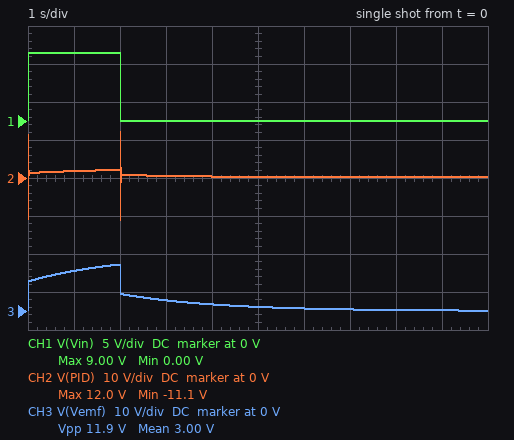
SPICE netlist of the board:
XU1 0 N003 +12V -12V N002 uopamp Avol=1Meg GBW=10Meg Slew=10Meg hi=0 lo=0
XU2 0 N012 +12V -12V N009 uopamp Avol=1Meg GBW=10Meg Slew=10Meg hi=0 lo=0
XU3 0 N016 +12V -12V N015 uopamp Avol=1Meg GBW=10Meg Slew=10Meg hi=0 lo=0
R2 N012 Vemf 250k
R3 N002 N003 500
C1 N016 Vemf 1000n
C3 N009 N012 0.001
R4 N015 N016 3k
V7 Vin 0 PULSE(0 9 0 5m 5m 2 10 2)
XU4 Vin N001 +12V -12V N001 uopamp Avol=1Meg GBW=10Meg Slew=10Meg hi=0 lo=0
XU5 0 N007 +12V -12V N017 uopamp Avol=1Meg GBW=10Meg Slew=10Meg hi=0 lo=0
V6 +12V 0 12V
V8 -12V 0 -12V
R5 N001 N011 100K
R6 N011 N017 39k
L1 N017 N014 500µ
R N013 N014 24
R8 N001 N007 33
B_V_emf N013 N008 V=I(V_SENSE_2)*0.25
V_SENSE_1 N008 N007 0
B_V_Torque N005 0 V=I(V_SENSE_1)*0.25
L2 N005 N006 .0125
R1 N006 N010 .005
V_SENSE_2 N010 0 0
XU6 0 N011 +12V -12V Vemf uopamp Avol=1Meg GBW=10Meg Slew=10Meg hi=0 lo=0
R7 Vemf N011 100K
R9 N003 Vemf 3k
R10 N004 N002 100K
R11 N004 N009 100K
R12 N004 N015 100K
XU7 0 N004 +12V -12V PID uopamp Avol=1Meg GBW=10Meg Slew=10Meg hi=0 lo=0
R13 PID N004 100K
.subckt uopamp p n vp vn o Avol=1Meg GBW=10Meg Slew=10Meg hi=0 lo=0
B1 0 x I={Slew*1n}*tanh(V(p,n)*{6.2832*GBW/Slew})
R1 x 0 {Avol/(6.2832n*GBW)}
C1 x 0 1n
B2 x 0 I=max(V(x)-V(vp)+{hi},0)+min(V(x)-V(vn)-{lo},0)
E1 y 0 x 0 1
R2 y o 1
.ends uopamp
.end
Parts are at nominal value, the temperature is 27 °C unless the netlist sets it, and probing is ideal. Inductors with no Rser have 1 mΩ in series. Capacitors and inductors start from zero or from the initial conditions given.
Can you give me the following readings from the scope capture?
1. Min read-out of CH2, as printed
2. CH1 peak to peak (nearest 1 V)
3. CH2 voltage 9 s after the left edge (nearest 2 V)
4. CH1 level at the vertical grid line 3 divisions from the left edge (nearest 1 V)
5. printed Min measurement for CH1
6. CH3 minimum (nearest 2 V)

-11.1 V
9 V
0 V
0 V
0.00 V
0 V
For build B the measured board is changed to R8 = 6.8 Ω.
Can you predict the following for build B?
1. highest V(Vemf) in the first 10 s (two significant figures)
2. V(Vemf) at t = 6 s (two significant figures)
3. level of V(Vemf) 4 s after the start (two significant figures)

12 V
1.4 V
3.7 V
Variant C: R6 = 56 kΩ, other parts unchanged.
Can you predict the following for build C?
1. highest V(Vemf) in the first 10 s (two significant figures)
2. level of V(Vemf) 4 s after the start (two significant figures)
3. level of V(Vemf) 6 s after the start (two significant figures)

5.8 V
1.2 V
460 mV
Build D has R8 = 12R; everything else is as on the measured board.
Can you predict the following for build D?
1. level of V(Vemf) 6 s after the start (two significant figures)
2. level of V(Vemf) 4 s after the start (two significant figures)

1.2 V
3.2 V
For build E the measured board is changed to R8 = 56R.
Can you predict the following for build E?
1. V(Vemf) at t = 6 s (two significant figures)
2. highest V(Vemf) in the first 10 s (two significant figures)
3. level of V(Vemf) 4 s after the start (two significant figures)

390 mV
3.5 V
1.0 V
